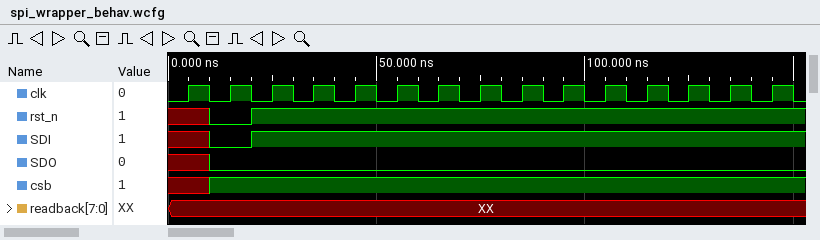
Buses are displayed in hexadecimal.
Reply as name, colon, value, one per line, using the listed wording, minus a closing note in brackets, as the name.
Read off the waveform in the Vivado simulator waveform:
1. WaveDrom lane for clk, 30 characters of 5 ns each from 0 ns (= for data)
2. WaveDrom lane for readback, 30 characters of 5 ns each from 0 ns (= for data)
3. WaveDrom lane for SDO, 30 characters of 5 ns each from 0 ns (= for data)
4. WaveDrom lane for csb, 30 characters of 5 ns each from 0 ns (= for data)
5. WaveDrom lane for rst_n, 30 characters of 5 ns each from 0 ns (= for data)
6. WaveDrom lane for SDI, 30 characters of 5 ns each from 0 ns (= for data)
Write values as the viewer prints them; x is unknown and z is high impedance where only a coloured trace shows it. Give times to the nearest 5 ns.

WaveDrom lane for clk, 30 characters of 5 ns each from 0 ns: {name: 'clk', wave: '010101010101010101010101010101'}
WaveDrom lane for readback, 30 characters of 5 ns each from 0 ns: {name: 'readback', wave: 'x.............................'}
WaveDrom lane for SDO, 30 characters of 5 ns each from 0 ns: {name: 'SDO', wave: 'x.0...........................'}
WaveDrom lane for csb, 30 characters of 5 ns each from 0 ns: {name: 'csb', wave: 'x.1...........................'}
WaveDrom lane for rst_n, 30 characters of 5 ns each from 0 ns: {name: 'rst_n', wave: 'x.0.1.........................'}
WaveDrom lane for SDI, 30 characters of 5 ns each from 0 ns: {name: 'SDI', wave: 'x.0.1.........................'}
